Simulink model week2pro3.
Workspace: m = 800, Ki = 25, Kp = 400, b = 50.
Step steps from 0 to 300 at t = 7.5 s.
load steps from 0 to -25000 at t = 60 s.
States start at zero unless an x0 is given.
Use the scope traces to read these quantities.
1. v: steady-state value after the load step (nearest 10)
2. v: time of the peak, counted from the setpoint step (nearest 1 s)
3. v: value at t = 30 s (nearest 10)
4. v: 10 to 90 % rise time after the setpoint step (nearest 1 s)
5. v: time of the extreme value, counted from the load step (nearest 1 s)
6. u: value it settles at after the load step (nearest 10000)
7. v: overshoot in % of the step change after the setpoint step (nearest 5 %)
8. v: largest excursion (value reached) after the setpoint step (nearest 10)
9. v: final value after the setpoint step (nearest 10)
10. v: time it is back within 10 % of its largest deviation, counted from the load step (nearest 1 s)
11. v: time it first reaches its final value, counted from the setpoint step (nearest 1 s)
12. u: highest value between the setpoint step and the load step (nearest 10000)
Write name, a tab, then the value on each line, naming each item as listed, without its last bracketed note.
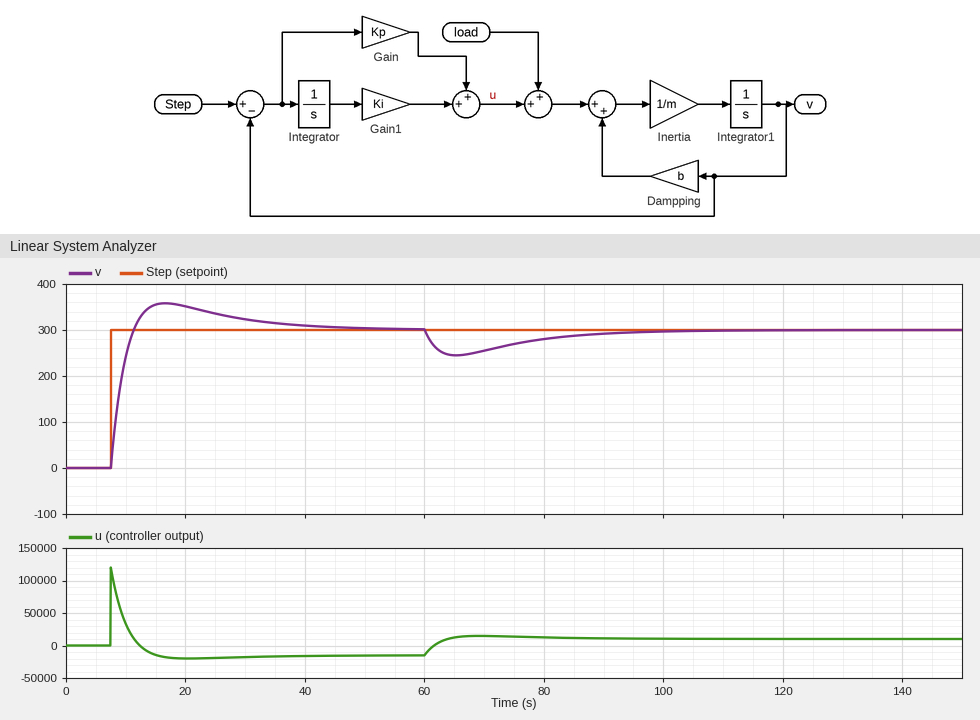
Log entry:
v: steady-state value after the load step	300
v: time of the peak, counted from the setpoint step	9 s
v: value at t = 30 s	320
v: 10 to 90 % rise time after the setpoint step	3 s
v: time of the extreme value, counted from the load step	5 s
u: value it settles at after the load step	10000
v: overshoot in % of the step change after the setpoint step	20 %
v: largest excursion (value reached) after the setpoint step	360
v: final value after the setpoint step	300
v: time it is back within 10 % of its largest deviation, counted from the load step	34 s
v: time it first reaches its final value, counted from the setpoint step	4 s
u: highest value between the setpoint step and the load step	120000
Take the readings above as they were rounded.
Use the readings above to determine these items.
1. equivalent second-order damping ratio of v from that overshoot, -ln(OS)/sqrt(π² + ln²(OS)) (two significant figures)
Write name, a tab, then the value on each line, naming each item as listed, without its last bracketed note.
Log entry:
equivalent second-order damping ratio of v from that overshoot, -ln(OS)/sqrt(π² + ln²(OS))	0.46
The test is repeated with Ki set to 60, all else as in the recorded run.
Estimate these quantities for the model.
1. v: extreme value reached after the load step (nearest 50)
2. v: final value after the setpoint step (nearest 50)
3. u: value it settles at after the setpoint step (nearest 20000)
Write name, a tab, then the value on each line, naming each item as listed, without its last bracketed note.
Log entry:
v: extreme value reached after the load step	250
v: final value after the setpoint step	300
u: value it settles at after the setpoint step	-20000
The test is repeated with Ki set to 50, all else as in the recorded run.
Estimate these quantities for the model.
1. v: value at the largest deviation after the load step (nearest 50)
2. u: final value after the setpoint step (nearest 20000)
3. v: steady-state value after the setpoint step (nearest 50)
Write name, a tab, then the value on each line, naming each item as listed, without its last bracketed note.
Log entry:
v: value at the largest deviation after the load step	250
u: final value after the setpoint step	-20000
v: steady-state value after the setpoint step	300
